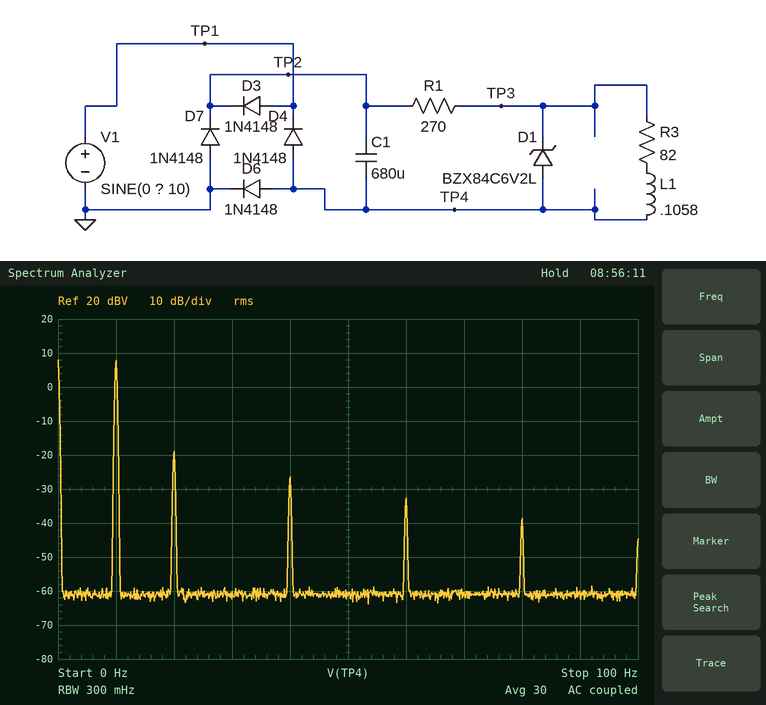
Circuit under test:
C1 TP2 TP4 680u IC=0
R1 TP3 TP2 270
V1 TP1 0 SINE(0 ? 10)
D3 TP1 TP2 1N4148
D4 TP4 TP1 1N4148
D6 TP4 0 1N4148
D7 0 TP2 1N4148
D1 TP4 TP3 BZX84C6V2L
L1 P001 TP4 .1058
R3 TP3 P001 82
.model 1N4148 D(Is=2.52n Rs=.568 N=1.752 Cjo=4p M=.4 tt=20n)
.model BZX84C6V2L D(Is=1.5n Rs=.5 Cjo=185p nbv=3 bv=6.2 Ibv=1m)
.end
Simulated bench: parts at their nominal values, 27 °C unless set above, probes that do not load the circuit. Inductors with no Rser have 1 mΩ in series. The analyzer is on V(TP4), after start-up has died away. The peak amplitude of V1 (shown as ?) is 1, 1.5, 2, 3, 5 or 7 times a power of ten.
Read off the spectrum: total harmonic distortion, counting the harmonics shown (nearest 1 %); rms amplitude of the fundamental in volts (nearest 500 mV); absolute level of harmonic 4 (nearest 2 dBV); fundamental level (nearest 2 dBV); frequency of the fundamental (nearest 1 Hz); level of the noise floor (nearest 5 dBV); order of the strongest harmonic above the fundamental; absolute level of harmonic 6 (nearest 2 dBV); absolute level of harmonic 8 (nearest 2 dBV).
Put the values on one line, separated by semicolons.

5 %; 2.5 V; -26 dBV; 8 dBV; 10 Hz; -60 dBV; 2; -32 dBV; -38 dBV
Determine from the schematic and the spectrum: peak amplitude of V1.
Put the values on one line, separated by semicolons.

7 V
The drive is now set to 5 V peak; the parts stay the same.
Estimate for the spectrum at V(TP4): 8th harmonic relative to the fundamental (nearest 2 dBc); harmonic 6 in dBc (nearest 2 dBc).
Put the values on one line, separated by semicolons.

-48 dBc; -42 dBc
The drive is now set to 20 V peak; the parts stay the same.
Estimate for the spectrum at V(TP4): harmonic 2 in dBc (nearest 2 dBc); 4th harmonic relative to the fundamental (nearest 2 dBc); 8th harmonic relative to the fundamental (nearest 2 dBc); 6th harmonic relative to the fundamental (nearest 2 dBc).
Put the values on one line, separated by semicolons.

-26 dBc; -32 dBc; -44 dBc; -38 dBc
